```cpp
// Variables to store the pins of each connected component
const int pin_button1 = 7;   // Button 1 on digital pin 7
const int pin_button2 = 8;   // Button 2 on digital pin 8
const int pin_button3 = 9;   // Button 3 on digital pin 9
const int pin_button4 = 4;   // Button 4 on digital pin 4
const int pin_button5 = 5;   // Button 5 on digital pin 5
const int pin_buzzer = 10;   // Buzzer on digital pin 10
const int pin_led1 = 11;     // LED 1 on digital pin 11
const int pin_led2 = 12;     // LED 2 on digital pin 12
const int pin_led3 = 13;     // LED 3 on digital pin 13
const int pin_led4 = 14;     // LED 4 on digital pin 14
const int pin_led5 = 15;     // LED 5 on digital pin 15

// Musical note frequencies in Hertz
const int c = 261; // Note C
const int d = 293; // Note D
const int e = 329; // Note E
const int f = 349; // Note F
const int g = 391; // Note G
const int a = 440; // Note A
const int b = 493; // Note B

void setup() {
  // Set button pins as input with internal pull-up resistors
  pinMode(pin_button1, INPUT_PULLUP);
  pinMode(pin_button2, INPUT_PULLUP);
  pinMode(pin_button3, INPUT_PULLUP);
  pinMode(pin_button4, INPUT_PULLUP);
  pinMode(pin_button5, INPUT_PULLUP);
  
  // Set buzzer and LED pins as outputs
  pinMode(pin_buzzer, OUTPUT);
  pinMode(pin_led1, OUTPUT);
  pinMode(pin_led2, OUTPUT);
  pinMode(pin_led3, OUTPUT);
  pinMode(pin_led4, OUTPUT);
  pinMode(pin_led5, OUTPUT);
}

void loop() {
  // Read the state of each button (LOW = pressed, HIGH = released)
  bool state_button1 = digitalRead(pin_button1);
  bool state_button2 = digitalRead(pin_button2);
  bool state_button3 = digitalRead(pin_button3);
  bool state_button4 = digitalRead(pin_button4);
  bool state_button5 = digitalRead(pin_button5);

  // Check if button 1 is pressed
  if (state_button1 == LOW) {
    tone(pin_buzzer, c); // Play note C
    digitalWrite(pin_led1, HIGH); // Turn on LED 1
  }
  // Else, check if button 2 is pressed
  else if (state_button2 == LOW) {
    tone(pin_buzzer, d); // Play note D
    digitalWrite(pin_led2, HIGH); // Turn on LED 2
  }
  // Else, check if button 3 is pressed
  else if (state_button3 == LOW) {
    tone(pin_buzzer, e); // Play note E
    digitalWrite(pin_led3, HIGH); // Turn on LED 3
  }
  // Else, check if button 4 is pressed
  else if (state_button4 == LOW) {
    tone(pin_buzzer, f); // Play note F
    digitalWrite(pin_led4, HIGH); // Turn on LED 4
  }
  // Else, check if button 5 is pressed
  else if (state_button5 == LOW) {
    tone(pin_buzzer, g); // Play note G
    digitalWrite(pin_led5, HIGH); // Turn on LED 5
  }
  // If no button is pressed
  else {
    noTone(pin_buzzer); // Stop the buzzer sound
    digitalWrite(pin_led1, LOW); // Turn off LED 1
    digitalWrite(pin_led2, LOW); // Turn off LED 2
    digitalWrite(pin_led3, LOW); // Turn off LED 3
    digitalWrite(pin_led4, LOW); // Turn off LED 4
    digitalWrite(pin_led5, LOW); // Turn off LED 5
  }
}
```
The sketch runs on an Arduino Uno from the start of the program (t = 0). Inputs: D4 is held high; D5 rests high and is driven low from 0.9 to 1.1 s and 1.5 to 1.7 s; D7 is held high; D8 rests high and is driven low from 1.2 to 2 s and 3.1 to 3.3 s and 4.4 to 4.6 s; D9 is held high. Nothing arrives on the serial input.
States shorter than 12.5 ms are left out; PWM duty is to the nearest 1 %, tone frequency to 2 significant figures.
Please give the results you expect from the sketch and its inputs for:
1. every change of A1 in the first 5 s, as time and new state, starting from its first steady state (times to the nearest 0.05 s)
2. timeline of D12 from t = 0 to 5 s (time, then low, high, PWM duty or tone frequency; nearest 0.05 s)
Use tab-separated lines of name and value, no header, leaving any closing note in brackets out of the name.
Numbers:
every change of A1 in the first 5 s, as time and new state, starting from its first steady state	0 s low; 0.9 s high; 1.1 s low
timeline of D12 from t = 0 to 5 s	0 s low; 1.2 s high; 2 s low; 3.1 s high; 3.3 s low; 4.4 s high; 4.6 s low
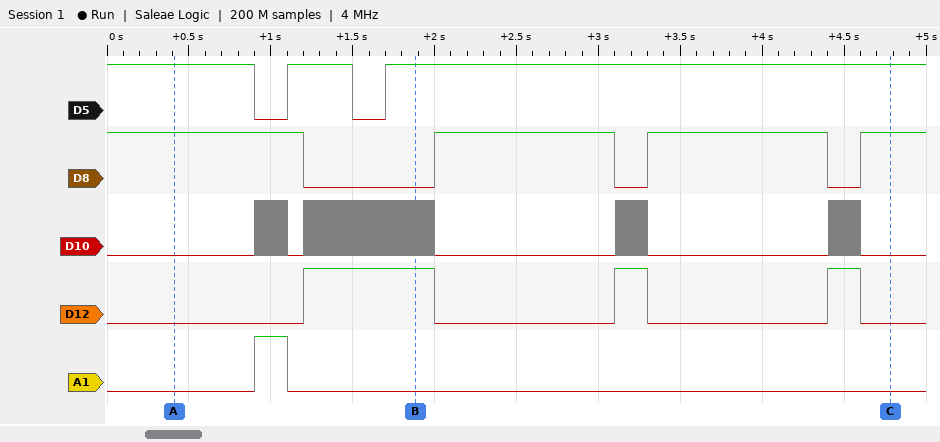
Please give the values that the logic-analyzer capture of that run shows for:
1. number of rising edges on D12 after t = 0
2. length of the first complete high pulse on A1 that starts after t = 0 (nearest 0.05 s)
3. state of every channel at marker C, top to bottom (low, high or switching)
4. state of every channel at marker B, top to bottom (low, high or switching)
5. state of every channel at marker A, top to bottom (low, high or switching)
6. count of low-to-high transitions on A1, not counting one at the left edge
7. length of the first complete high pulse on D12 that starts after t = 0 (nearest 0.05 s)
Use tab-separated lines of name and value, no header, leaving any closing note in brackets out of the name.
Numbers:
number of rising edges on D12 after t = 0	3
length of the first complete high pulse on A1 that starts after t = 0	0.20 s
state of every channel at marker C, top to bottom	D5 high, D8 high, D10 low, D12 low, A1 low
state of every channel at marker B, top to bottom	D5 high, D8 low, D10 switching, D12 high, A1 low
state of every channel at marker A, top to bottom	D5 high, D8 high, D10 low, D12 low, A1 low
count of low-to-high transitions on A1, not counting one at the left edge	1
length of the first complete high pulse on D12 that starts after t = 0	0.80 s
